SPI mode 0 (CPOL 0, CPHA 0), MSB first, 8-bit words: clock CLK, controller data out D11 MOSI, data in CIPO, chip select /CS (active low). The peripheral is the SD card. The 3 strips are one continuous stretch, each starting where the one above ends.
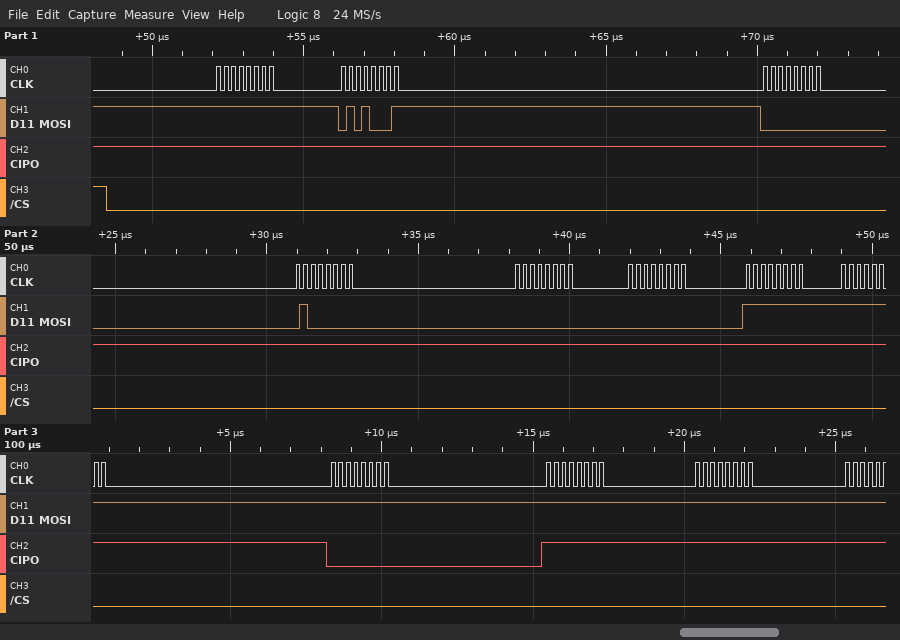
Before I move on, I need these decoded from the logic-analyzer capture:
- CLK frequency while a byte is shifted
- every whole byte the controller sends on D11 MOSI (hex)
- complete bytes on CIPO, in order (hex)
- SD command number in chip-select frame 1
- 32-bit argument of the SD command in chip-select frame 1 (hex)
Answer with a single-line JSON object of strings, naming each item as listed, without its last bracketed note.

{"CLK frequency while a byte is shifted": "4 MHz", "every whole byte the controller sends on D11 MOSI": "0xFF 0x51 0x00 0x40 0x00 0x00 0xFF 0xFF 0xFF 0xFF 0xFF", "complete bytes on CIPO, in order": "0xFF 0xFF 0xFF 0xFF 0xFF 0xFF 0xFF 0xFF 0x00 0xFF 0xFF", "SD command number in chip-select frame 1": "CMD17", "32-bit argument of the SD command in chip-select frame 1": "0x00400000"}
